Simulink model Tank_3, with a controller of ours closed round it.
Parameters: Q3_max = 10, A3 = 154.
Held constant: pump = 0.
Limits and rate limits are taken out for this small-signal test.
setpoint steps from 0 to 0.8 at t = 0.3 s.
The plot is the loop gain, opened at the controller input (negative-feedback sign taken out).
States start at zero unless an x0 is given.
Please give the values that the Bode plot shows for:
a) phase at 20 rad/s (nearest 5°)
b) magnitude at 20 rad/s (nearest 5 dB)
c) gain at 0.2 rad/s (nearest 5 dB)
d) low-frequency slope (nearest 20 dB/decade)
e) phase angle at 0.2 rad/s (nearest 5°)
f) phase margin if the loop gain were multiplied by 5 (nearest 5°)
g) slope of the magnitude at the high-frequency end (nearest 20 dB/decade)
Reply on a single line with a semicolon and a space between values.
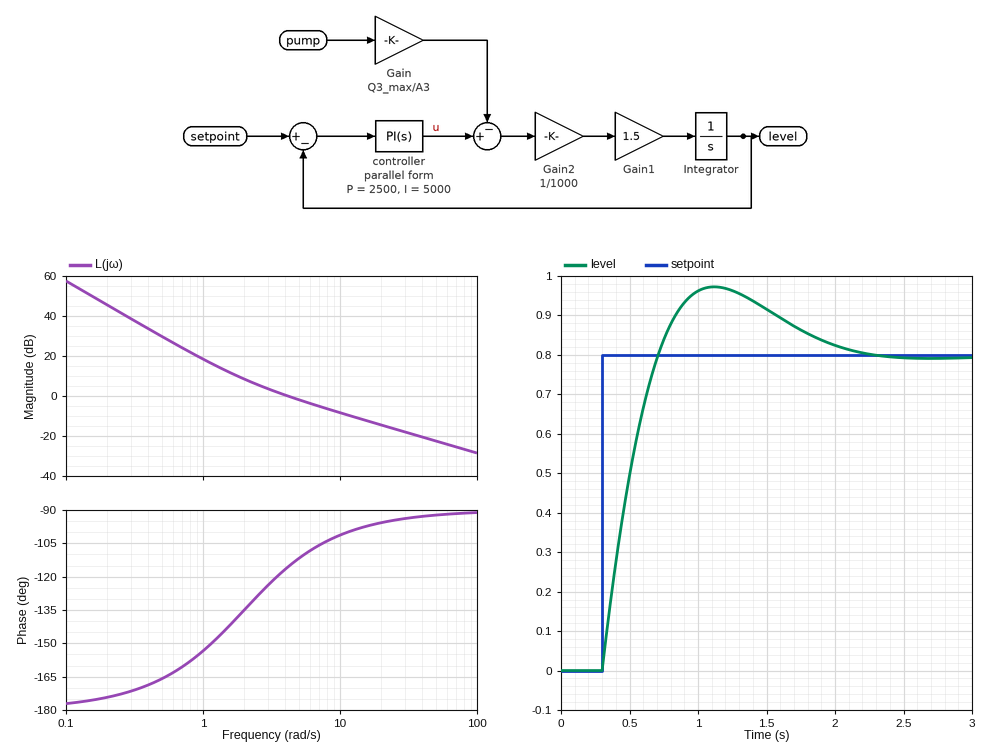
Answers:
-95°; -15 dB; 45 dB; -40 dB/decade; -175°; 85°; -20 dB/decade
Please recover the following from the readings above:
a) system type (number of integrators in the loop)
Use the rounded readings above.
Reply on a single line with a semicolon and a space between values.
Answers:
2
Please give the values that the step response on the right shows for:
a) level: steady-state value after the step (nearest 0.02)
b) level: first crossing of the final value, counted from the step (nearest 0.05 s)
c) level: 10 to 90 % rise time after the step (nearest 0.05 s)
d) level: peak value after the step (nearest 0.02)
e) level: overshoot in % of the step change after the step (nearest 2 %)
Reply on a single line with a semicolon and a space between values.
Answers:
0.80; 0.40 s; 0.30 s; 0.98; 22 %
